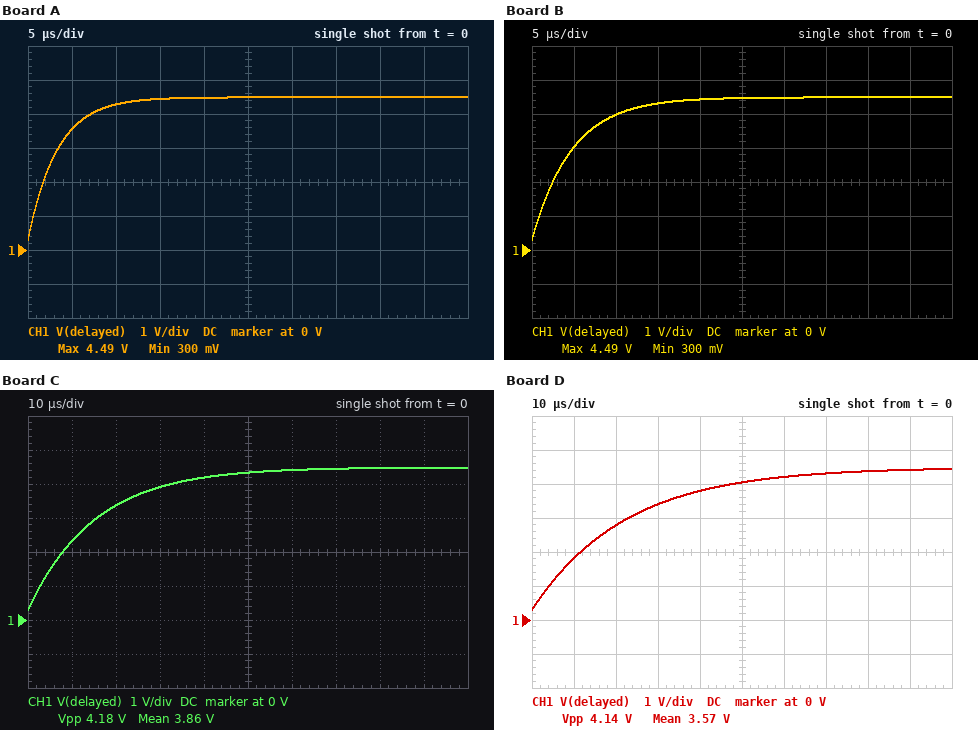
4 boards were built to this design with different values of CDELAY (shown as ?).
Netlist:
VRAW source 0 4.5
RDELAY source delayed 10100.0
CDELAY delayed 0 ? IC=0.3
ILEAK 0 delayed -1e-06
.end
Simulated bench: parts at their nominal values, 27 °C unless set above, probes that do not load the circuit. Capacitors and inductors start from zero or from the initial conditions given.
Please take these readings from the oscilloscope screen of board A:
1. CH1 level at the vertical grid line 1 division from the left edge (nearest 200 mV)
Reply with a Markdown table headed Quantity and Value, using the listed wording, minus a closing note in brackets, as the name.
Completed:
| Quantity | Value |
|---|---|
| CH1 level at the vertical grid line 1 division from the left edge | 3.6 V |
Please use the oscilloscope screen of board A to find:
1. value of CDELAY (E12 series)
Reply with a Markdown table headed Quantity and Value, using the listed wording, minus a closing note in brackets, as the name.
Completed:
| Quantity | Value |
|---|---|
| value of CDELAY | 330 pF |
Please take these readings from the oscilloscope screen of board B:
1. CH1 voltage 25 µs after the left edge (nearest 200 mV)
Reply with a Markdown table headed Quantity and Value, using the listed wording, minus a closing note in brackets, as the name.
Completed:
| Quantity | Value |
|---|---|
| CH1 voltage 25 µs after the left edge | 4.4 V |
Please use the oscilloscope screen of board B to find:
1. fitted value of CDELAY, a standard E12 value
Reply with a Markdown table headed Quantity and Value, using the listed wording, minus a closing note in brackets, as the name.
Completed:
| Quantity | Value |
|---|---|
| fitted value of CDELAY, a standard E12 value | 470 pF |
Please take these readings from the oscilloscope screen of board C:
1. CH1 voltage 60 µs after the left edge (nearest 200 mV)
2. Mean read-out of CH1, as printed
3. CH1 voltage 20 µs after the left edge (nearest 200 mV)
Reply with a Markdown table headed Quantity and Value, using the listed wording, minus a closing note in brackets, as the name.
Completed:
| Quantity | Value |
|---|---|
| CH1 voltage 60 µs after the left edge | 4.4 V |
| Mean read-out of CH1, as printed | 3.86 V |
| CH1 voltage 20 µs after the left edge | 3.4 V |
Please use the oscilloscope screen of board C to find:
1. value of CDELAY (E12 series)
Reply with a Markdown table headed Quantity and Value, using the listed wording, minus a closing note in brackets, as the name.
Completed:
| Quantity | Value |
|---|---|
| value of CDELAY | 1.5 nF |
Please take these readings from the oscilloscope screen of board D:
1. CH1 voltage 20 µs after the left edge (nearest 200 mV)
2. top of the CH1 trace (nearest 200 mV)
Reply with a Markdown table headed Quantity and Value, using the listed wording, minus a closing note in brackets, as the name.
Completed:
| Quantity | Value |
|---|---|
| CH1 voltage 20 µs after the left edge | 2.8 V |
| top of the CH1 trace | 4.4 V |
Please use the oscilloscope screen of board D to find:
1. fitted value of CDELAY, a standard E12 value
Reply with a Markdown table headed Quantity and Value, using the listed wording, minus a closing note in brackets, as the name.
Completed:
| Quantity | Value |
|---|---|
| fitted value of CDELAY, a standard E12 value | 2.2 nF |
